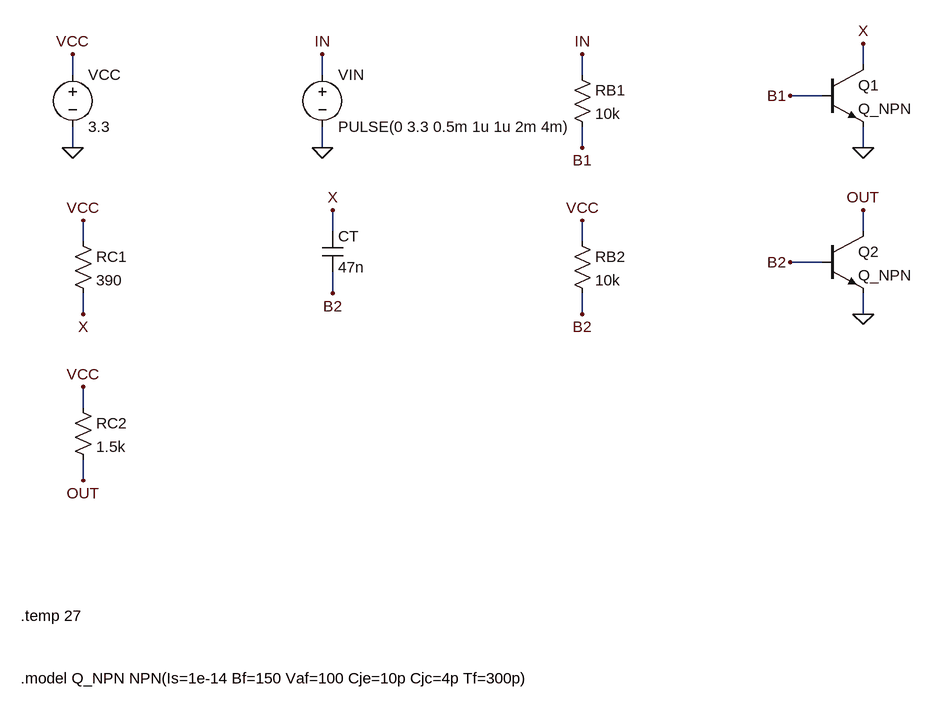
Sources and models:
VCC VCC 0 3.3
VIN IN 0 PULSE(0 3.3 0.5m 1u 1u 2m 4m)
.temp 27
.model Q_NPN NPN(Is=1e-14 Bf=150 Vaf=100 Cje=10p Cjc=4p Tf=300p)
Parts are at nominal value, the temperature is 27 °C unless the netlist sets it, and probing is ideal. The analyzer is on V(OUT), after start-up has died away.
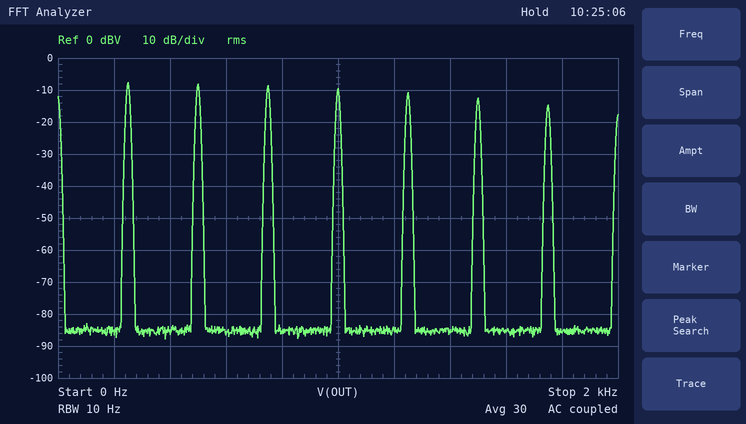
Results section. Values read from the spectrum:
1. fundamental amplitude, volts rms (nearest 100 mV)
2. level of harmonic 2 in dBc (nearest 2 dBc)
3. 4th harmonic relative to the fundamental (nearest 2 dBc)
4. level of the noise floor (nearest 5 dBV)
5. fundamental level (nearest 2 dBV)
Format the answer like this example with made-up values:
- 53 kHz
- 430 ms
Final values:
- 400 mV
- 0 dBc
- -2 dBc
- -85 dBV
- -8 dBV
